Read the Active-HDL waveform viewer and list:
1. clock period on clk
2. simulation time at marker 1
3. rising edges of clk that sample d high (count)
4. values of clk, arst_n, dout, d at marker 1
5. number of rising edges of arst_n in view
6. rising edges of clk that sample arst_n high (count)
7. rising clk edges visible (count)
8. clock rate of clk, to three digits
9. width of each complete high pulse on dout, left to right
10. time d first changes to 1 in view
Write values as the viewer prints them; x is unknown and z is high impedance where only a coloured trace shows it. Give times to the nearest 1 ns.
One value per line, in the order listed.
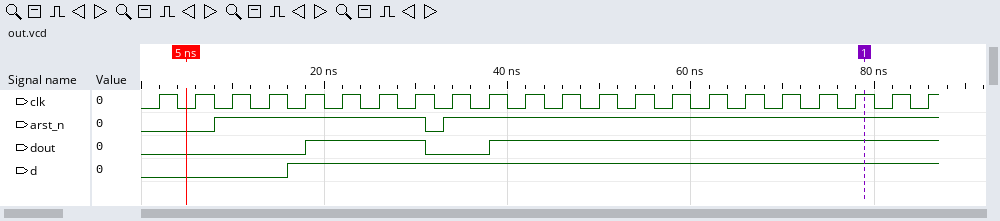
4 ns
79 ns
18
clk=1, arst_n=1, dout=1, d=1
2
20
22
250 MHz
13 ns
16 ns
